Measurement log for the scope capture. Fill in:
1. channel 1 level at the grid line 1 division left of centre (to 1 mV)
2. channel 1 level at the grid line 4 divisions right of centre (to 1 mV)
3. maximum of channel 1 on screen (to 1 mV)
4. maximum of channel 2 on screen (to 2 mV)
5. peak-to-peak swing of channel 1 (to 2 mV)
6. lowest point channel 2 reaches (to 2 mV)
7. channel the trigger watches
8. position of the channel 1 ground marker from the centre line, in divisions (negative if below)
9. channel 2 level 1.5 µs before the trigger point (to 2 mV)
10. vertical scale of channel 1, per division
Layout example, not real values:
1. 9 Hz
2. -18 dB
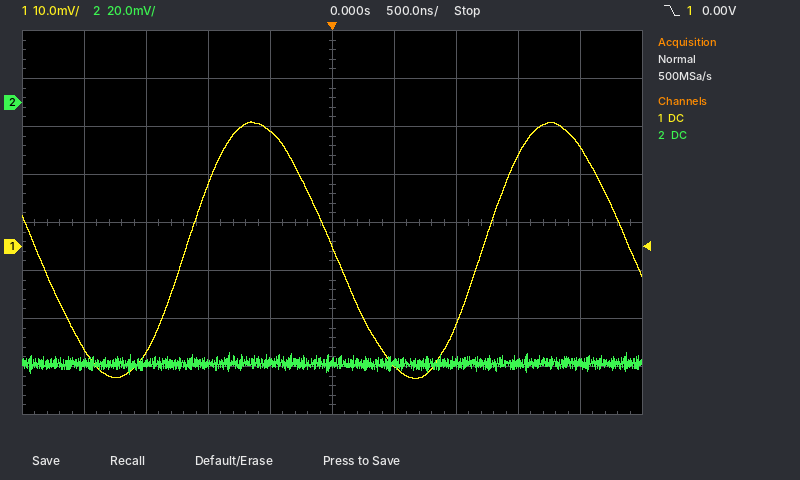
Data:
1. 24 mV
2. 21 mV
3. 26 mV
4. -104 mV
5. 54 mV
6. -114 mV
7. channel 1
8. -0.5 div
9. -108 mV
10. 10 mV
